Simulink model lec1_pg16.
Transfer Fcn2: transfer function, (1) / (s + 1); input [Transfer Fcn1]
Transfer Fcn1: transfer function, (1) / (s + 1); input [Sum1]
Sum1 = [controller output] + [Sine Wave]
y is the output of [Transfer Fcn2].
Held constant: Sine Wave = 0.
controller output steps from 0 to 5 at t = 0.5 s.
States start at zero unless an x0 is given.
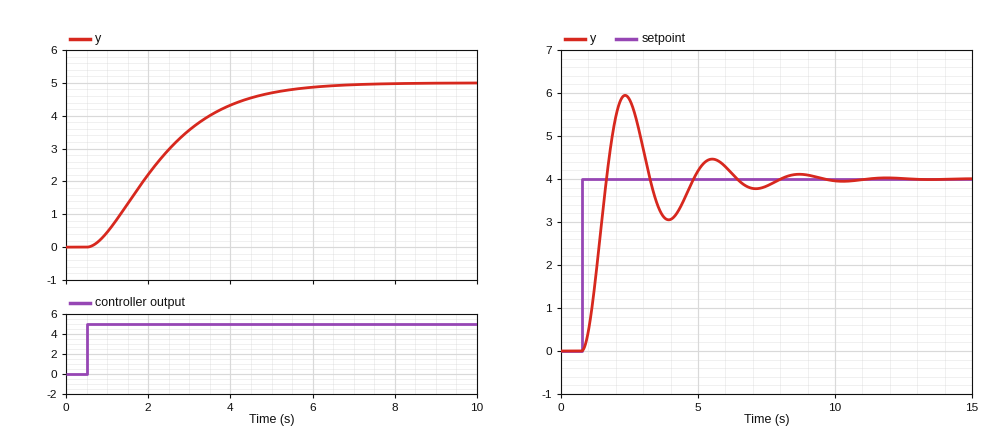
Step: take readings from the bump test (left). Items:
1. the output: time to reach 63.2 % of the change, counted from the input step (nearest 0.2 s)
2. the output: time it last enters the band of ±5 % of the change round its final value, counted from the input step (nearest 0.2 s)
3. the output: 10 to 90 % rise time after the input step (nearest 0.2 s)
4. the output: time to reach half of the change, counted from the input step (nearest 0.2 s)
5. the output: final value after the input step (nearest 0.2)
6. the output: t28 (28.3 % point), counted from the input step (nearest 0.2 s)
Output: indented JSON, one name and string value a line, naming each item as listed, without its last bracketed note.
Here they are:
{
  "the output: time to reach 63.2 % of the change, counted from the input step": "2.2 s",
  "the output: time it last enters the band of ±5 % of the change round its final value, counted from the input step": "4.8 s",
  "the output: 10 to 90 % rise time after the input step": "3.4 s",
  "the output: time to reach half of the change, counted from the input step": "1.6 s",
  "the output: final value after the input step": "5.0",
  "the output: t28 (28.3 % point), counted from the input step": "1.0 s"
}
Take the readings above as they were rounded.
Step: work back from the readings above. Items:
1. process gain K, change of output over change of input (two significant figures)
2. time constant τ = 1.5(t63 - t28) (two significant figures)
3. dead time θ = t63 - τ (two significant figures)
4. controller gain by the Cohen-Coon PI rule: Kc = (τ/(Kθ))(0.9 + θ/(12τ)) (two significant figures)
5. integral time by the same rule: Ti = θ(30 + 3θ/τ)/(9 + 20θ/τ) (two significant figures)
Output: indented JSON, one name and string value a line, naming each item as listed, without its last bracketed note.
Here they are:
{
  "process gain K, change of output over change of input": "1.0",
  "time constant τ = 1.5(t63 - t28)": "1.8 s",
  "dead time θ = t63 - τ": "0.40 s",
  "controller gain by the Cohen-Coon PI rule: Kc = (τ/(Kθ))(0.9 + θ/(12τ))": "4.1",
  "integral time by the same rule: Ti = θ(30 + 3θ/τ)/(9 + 20θ/τ)": "0.91 s"
}
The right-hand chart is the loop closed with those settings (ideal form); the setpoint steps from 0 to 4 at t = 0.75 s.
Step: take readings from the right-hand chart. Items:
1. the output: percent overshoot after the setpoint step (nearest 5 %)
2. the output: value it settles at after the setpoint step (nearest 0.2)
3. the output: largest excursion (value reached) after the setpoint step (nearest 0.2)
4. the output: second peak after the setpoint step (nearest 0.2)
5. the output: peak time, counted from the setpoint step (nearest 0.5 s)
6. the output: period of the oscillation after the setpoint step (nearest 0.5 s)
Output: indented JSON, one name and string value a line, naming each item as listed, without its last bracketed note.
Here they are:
{
  "the output: percent overshoot after the setpoint step": "50 %",
  "the output: value it settles at after the setpoint step": "4.0",
  "the output: largest excursion (value reached) after the setpoint step": "6.0",
  "the output: second peak after the setpoint step": "4.4",
  "the output: peak time, counted from the setpoint step": "1.5 s",
  "the output: period of the oscillation after the setpoint step": "3.0 s"
}
